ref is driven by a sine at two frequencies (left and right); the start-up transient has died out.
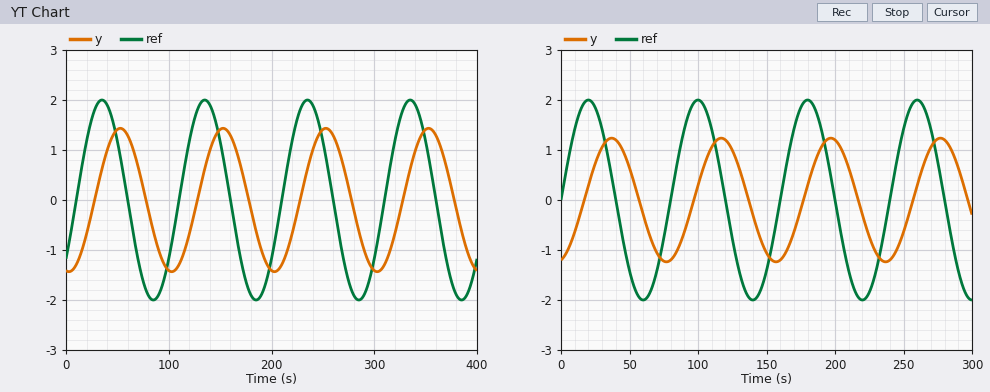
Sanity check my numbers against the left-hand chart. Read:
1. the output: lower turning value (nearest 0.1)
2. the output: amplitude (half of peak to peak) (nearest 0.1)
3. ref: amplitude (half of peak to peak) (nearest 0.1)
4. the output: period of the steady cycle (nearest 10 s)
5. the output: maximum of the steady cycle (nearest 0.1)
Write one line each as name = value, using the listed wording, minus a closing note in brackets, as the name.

the output: lower turning value = -1.4
the output: amplitude (half of peak to peak) = 1.4
ref: amplitude (half of peak to peak) = 2.0
the output: period of the steady cycle = 100 s
the output: maximum of the steady cycle = 1.4
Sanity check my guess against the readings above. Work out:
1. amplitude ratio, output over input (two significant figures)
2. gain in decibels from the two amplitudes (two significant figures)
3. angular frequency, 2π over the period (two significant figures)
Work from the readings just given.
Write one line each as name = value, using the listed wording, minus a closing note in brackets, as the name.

amplitude ratio, output over input = 0.70
gain in decibels from the two amplitudes = -3.1 dB
angular frequency, 2π over the period = 0.063 rad/s
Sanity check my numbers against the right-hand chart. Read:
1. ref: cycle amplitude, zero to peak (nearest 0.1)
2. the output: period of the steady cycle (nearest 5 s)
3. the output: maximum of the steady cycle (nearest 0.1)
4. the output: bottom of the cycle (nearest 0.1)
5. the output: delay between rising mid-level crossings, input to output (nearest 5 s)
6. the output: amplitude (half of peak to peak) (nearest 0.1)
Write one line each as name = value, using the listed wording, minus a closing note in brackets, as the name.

ref: cycle amplitude, zero to peak = 2.0
the output: period of the steady cycle = 80 s
the output: maximum of the steady cycle = 1.2
the output: bottom of the cycle = -1.2
the output: delay between rising mid-level crossings, input to output = 15 s
the output: amplitude (half of peak to peak) = 1.2
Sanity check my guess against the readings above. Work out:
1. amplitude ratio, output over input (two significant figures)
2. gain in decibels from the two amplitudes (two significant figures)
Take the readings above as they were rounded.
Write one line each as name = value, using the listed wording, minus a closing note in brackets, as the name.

amplitude ratio, output over input = 0.60
gain in decibels from the two amplitudes = -4.4 dB
